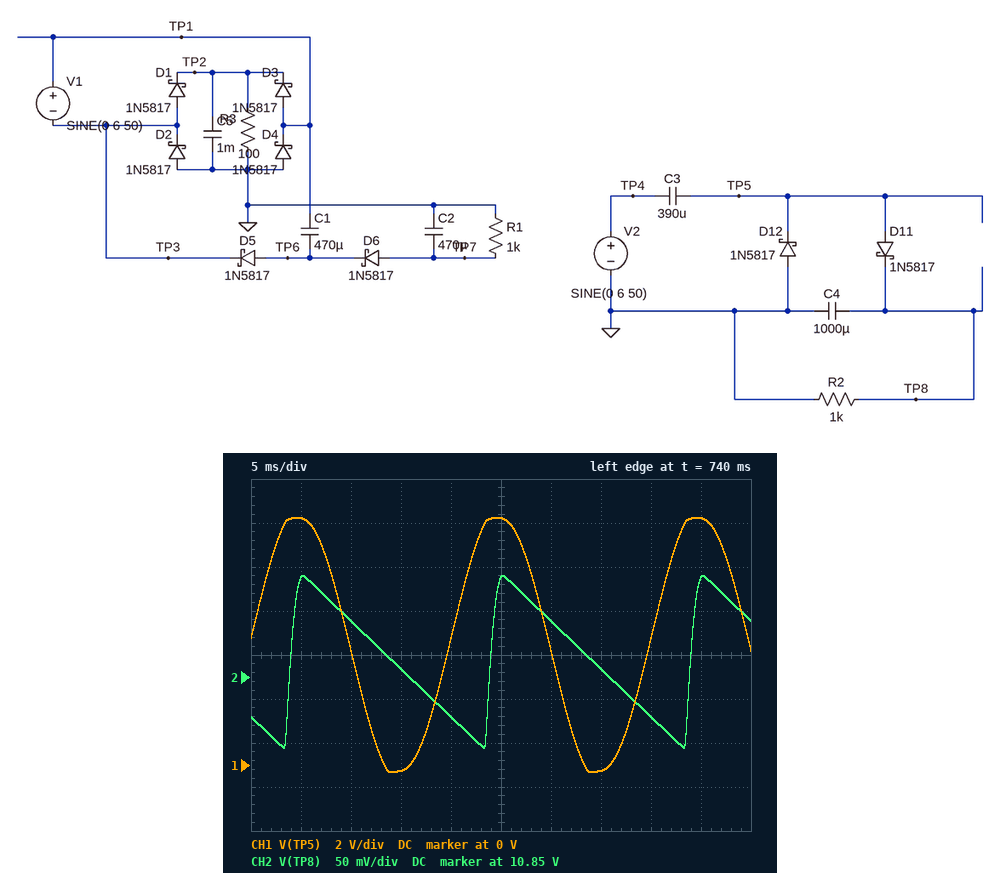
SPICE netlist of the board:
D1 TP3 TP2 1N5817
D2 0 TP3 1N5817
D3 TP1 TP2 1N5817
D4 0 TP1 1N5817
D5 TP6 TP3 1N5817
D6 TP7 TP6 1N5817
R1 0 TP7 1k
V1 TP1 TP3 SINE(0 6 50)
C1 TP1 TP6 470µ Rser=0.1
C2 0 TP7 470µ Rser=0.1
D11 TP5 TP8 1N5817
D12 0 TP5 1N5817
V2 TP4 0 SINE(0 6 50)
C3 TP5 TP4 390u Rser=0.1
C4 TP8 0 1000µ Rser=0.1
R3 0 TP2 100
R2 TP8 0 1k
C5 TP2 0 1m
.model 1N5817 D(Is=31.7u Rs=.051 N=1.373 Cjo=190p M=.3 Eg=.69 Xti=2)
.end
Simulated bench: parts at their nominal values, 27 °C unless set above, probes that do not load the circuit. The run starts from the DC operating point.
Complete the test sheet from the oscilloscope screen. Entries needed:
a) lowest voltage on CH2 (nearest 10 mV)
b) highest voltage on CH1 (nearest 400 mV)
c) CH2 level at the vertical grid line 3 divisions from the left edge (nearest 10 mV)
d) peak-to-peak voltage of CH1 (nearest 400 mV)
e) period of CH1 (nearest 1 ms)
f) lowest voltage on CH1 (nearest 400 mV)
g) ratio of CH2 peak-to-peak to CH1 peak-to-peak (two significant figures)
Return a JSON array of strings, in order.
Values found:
["10.77 V", "11.2 V", "10.86 V", "11.6 V", "20 ms", "-400 mV", "0.017"]
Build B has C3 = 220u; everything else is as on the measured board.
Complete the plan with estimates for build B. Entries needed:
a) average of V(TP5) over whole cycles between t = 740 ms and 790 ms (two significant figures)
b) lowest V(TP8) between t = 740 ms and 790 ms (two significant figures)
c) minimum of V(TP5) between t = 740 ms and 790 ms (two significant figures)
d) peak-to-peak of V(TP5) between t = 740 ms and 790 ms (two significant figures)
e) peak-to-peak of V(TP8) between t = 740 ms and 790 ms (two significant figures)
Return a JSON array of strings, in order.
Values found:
["5.3 V", "10 V", "-320 mV", "11 V", "190 mV"]
